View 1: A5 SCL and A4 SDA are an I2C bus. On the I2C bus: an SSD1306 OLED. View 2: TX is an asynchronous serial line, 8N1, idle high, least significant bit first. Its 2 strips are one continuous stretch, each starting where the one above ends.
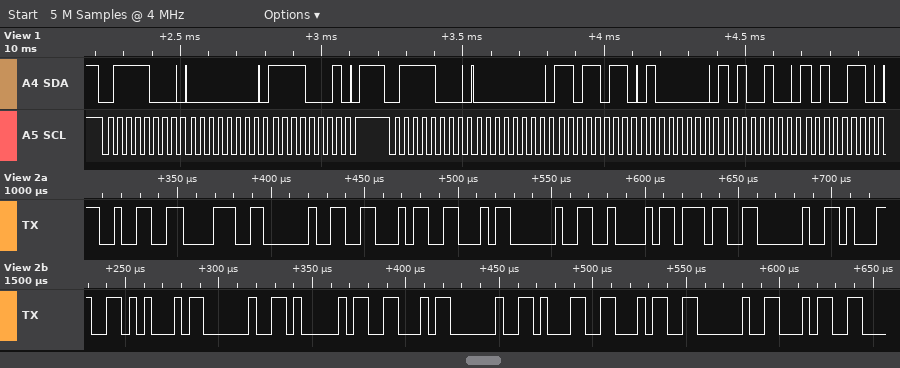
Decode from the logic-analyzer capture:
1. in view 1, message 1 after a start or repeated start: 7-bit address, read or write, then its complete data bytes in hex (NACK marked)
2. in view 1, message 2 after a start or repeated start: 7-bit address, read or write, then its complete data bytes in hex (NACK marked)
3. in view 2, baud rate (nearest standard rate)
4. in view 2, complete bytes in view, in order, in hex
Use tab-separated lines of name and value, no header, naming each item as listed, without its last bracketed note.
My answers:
in view 1, message 1 after a start or repeated start: 7-bit address, read or write, then its complete data bytes in hex	0x3C write: 00 F1
in view 1, message 2 after a start or repeated start: 7-bit address, read or write, then its complete data bytes in hex	0x3C write: 00 DB 40 A4 A6
in view 2, baud rate	250000 baud
in view 2, complete bytes in view, in order, in hex	32 38 20 46 46 20 42 37 20 31 45 20 41 46 20 31 34 20 34
